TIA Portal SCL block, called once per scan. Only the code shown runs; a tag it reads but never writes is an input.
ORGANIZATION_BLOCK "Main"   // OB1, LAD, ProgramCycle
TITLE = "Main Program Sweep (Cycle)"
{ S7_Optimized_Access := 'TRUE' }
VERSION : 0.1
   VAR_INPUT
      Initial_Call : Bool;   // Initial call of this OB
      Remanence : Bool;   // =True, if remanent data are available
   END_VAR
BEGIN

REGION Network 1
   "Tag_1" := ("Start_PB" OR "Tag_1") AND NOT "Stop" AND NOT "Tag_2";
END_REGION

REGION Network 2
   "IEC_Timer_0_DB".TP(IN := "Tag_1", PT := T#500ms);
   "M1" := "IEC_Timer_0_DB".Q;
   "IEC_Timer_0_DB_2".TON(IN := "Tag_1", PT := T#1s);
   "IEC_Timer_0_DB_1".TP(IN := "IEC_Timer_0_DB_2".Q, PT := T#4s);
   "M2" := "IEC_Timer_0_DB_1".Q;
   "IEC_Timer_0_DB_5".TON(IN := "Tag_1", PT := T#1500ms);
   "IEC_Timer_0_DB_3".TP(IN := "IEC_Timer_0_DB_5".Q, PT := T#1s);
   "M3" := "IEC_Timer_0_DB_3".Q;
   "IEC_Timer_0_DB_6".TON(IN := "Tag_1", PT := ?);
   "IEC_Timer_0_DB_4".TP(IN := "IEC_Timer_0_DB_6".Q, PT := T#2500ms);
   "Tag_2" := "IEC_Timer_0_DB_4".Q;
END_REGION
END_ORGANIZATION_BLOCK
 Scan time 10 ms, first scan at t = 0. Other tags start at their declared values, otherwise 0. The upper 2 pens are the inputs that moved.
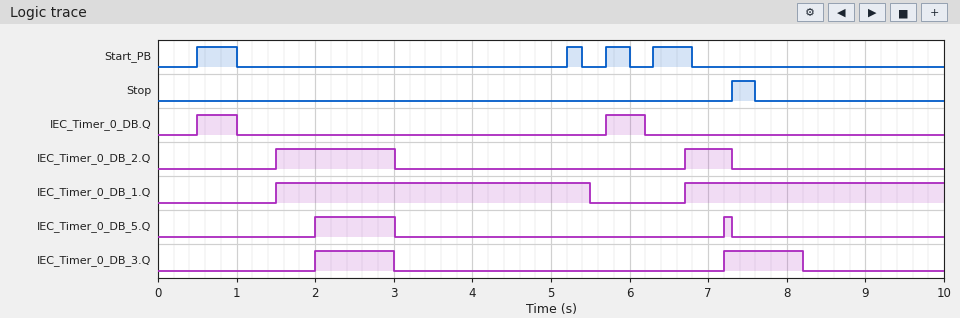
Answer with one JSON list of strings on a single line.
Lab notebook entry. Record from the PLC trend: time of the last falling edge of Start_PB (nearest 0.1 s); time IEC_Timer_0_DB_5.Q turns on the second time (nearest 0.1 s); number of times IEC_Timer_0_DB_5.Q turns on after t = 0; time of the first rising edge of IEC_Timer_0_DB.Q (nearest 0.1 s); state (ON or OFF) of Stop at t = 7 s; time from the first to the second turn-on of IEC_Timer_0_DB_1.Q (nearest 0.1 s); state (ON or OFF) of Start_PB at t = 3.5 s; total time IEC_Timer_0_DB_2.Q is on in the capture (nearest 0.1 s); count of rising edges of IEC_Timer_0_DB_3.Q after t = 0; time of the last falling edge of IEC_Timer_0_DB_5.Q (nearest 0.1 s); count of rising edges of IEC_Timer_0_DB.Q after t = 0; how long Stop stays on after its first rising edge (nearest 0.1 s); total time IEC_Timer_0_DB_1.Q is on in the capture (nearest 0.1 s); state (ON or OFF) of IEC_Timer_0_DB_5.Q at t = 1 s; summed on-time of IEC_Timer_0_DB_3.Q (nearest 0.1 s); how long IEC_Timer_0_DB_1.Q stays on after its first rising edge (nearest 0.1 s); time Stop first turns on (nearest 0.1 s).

["6.8 s", "7.2 s", "2", "0.5 s", "OFF", "5.2 s", "OFF", "2.1 s", "2", "7.3 s", "2", "0.3 s", "7.3 s", "OFF", "2.0 s", "4.0 s", "7.3 s"]
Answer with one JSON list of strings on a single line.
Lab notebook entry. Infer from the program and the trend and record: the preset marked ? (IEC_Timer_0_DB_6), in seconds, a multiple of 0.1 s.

["2.5 s"]
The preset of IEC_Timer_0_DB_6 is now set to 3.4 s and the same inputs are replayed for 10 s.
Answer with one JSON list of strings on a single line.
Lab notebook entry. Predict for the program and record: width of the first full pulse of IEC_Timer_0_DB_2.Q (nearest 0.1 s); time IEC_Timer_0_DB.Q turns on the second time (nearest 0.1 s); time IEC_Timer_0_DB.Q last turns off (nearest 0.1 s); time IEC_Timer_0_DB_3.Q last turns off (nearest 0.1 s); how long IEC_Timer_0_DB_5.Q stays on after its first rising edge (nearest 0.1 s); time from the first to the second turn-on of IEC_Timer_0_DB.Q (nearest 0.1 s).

["2.4 s", "6.4 s", "6.9 s", "3.0 s", "1.9 s", "5.9 s"]
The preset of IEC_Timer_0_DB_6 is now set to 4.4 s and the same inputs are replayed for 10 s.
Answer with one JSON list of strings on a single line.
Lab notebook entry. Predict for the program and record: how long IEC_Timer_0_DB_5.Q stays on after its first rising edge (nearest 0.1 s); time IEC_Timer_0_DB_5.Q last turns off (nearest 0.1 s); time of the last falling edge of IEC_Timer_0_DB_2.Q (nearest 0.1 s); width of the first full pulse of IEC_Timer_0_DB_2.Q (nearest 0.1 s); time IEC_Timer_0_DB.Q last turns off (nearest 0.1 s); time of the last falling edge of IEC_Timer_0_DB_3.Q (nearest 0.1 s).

["2.9 s", "4.9 s", "4.9 s", "3.4 s", "1.0 s", "3.0 s"]
